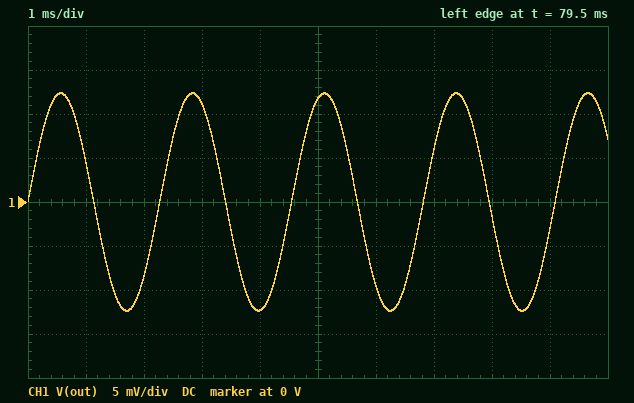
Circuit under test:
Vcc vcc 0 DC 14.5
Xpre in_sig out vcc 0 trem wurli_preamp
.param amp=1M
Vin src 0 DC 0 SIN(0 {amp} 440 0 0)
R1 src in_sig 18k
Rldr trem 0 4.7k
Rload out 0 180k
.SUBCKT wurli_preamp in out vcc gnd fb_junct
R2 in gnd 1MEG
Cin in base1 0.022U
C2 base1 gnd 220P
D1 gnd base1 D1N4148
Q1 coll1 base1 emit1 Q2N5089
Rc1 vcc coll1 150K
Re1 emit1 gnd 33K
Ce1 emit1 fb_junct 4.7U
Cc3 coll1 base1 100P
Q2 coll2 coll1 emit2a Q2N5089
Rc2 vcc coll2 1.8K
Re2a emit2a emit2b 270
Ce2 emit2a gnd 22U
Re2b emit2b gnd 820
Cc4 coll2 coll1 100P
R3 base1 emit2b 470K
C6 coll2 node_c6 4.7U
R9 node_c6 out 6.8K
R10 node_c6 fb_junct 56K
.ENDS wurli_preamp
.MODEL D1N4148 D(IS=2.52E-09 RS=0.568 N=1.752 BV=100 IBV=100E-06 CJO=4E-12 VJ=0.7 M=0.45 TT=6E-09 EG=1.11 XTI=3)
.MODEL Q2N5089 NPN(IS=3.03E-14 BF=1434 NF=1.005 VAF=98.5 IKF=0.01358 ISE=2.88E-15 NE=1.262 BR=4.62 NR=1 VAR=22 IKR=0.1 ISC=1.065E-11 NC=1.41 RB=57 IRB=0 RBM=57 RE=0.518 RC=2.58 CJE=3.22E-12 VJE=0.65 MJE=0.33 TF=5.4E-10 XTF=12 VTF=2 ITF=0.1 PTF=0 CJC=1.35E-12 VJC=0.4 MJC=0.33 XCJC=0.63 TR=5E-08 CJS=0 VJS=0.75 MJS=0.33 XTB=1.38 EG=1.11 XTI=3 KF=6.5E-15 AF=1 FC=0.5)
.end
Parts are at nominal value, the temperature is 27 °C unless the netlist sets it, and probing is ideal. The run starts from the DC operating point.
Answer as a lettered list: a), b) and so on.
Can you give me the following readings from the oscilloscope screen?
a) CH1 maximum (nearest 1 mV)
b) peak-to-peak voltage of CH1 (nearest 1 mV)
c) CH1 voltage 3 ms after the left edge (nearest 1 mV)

a) 12 mV
b) 25 mV
c) 11 mV
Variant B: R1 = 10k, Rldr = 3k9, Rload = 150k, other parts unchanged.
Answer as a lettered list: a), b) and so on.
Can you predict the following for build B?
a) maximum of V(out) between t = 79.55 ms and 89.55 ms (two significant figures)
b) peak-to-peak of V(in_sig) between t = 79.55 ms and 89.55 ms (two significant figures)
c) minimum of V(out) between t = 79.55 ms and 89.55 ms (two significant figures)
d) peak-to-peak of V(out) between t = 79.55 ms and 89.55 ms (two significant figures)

a) 15 mV
b) 1.9 mV
c) -15 mV
d) 29 mV
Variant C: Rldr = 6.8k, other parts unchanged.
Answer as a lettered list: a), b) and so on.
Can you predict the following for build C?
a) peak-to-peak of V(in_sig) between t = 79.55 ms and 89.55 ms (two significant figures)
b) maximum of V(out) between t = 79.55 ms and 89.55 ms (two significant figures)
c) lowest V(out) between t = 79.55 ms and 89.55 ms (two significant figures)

a) 1.9 mV
b) 9.3 mV
c) -9.3 mV
